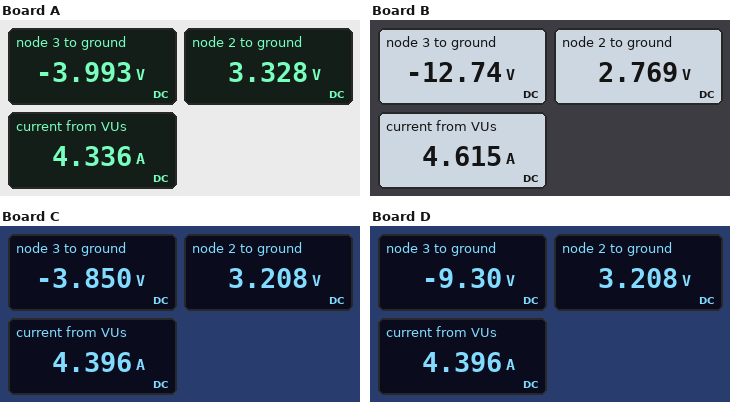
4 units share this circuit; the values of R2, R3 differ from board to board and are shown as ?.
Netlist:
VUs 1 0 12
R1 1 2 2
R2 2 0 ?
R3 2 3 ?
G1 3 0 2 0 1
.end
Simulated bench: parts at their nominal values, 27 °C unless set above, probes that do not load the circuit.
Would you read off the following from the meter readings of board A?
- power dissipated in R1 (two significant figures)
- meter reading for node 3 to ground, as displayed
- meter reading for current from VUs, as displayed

38 W
-3.993 V
4.336 A
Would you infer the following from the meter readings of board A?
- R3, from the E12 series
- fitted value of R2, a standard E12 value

2.2 Ω
3.3 Ω
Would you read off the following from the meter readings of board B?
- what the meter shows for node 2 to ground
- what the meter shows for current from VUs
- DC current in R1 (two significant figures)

2.769 V
4.615 A
4.6 A
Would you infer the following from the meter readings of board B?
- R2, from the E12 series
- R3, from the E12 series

1.5 Ω
5.6 Ω
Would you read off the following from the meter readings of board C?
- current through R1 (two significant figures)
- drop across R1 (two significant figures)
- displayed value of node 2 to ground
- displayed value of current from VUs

4.4 A
8.8 V
3.208 V
4.396 A
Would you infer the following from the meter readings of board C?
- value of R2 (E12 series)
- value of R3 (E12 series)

2.7 Ω
2.2 Ω
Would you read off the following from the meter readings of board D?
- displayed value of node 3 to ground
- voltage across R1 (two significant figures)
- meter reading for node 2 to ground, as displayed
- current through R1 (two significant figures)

-9.30 V
8.8 V
3.208 V
4.4 A
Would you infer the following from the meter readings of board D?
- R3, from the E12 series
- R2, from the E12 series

3.9 Ω
2.7 Ω
